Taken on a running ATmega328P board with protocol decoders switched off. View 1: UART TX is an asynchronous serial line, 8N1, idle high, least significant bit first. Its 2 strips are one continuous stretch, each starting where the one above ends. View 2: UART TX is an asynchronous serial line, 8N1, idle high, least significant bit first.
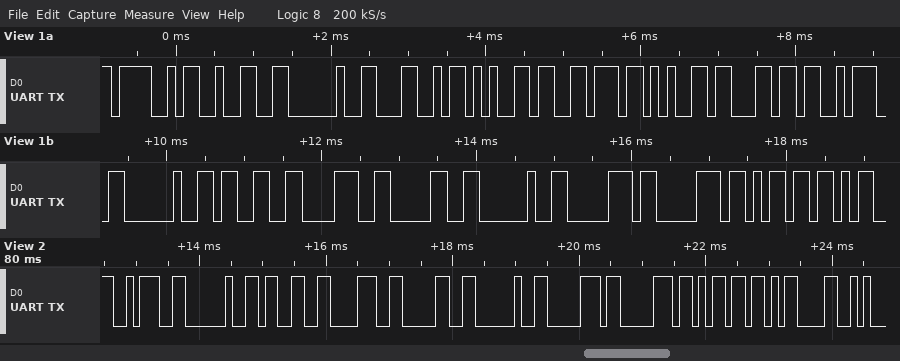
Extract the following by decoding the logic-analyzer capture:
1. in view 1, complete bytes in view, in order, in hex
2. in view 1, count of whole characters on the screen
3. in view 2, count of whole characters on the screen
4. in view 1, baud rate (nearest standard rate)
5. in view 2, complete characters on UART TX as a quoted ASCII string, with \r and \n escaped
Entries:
0x4F 0x32 0x20 0x4C 0x65 0x76 0x65 0x6C 0x3A 0x20 0x33 0x38 0x30 0x20 0x70 0x70 0x6D
17
10
9600 baud
": 380 ppm\r"
